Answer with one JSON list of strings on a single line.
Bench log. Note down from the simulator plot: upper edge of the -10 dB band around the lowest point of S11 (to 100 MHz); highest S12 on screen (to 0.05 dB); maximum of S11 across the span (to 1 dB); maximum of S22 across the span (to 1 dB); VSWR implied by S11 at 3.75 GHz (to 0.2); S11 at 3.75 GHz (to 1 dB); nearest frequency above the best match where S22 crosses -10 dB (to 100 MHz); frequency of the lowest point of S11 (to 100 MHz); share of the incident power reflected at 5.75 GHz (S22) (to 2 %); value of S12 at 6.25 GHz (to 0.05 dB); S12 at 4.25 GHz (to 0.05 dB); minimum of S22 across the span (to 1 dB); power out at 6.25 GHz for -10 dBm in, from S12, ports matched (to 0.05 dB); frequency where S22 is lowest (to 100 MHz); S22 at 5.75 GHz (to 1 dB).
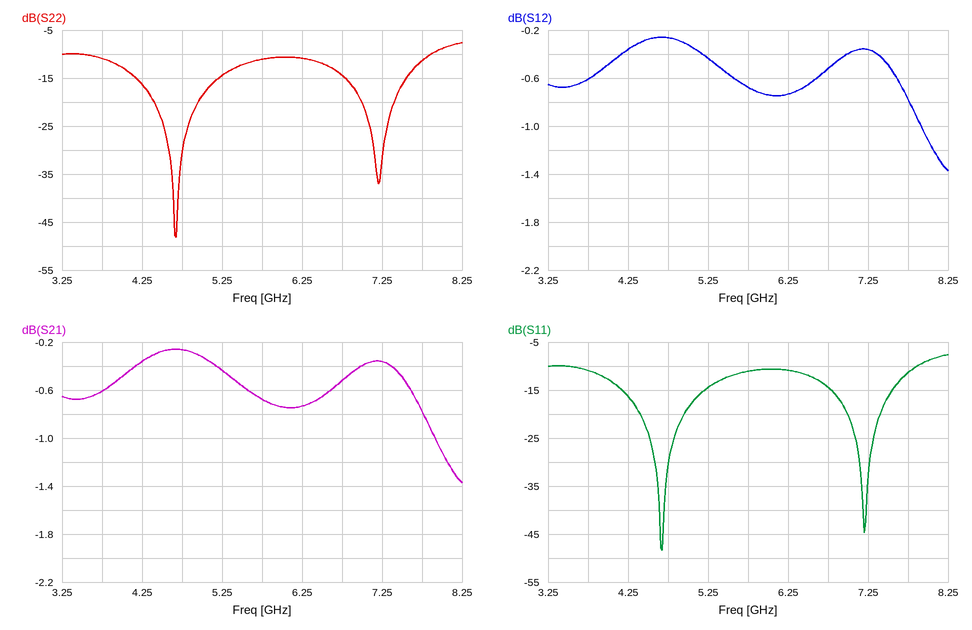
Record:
["7.9 GHz", "-0.25 dB", "-8 dB", "-8 dB", "1.8", "-11 dB", "7.9 GHz", "4.7 GHz", "8 %", "-0.75 dB", "-0.35 dB", "-48 dB", "-10.75 dBm", "4.7 GHz", "-11 dB"]
